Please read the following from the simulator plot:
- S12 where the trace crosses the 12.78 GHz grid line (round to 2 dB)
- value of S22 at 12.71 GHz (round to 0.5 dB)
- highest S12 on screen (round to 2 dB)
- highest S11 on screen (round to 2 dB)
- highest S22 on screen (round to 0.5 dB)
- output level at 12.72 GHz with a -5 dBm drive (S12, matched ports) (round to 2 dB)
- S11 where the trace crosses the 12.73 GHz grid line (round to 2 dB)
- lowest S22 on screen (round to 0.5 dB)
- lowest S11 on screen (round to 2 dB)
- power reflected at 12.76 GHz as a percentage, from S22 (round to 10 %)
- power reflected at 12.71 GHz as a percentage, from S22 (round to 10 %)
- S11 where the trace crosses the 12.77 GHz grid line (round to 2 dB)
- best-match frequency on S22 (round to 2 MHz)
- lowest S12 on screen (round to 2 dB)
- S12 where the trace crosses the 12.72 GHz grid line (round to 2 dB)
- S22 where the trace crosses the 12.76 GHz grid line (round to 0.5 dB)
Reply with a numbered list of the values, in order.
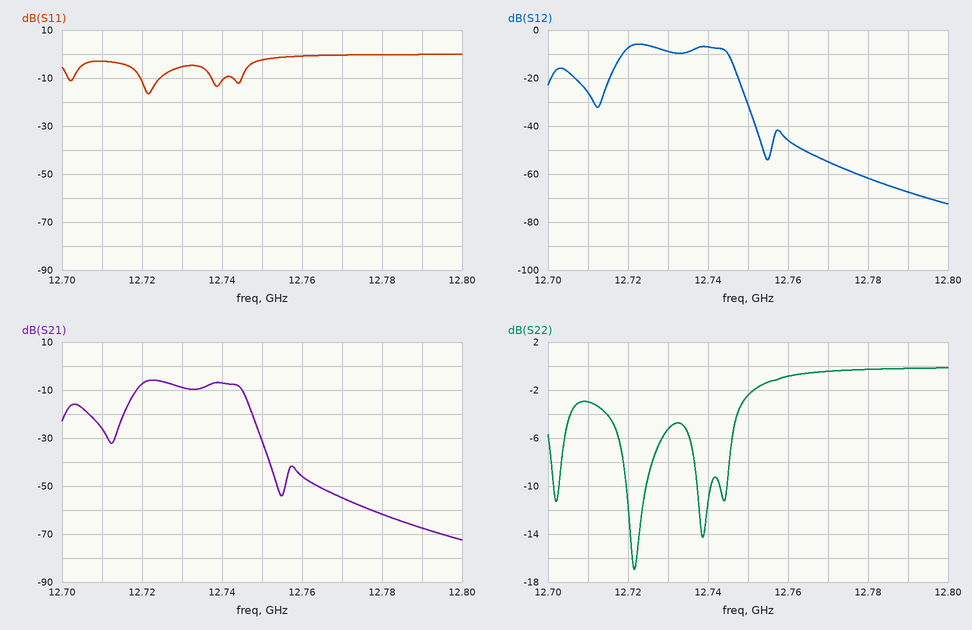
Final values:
1. -62 dB
2. -3.0 dB
3. -6 dB
4. 0 dB
5. 0.0 dB
6. -12 dBm
7. -6 dB
8. -17.0 dB
9. -16 dB
10. 80 %
11. 50 %
12. 0 dB
13. 12.722 GHz
14. -72 dB
15. -8 dB
16. -1.0 dB
